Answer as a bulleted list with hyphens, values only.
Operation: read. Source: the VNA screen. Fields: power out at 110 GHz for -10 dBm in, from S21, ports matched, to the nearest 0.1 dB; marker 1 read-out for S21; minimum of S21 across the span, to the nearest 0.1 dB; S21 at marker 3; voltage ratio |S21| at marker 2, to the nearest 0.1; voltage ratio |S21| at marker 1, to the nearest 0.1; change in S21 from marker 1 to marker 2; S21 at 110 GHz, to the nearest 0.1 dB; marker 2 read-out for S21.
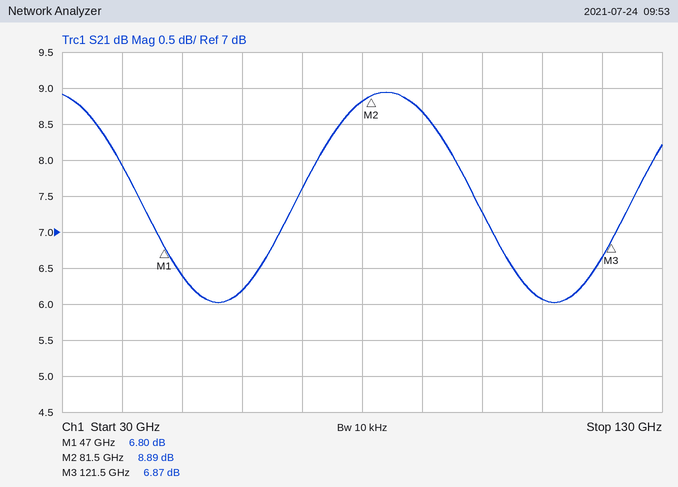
- -3.9 dBm
- 6.80 dB
- 6.0 dB
- 6.87 dB
- 2.8
- 2.2
- 2.09 dB
- 6.1 dB
- 8.89 dB
